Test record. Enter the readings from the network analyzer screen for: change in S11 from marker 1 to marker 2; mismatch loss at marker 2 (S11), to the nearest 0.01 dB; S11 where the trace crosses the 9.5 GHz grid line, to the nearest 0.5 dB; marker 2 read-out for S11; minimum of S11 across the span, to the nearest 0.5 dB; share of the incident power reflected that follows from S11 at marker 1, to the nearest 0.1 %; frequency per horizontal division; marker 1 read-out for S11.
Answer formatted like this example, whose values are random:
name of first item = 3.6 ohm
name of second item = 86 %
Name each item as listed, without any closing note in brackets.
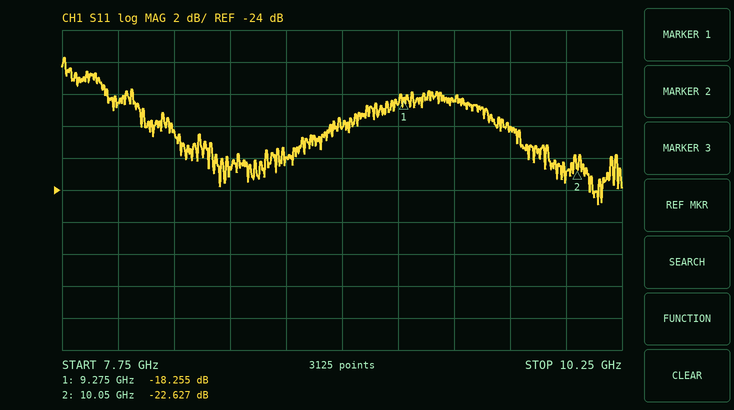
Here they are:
change in S11 from marker 1 to marker 2 = -4.372 dB
mismatch loss at marker 2 (S11), to the nearest 0.01 dB = 0.02 dB
S11 where the trace crosses the 9.5 GHz grid line, to the nearest 0.5 dB = -18.5 dB
marker 2 read-out for S11 = -22.627 dB
minimum of S11 across the span, to the nearest 0.5 dB = -25.0 dB
share of the incident power reflected that follows from S11 at marker 1, to the nearest 0.1 % = 1.5 %
frequency per horizontal division = 250 MHz
marker 1 read-out for S11 = -18.255 dB
